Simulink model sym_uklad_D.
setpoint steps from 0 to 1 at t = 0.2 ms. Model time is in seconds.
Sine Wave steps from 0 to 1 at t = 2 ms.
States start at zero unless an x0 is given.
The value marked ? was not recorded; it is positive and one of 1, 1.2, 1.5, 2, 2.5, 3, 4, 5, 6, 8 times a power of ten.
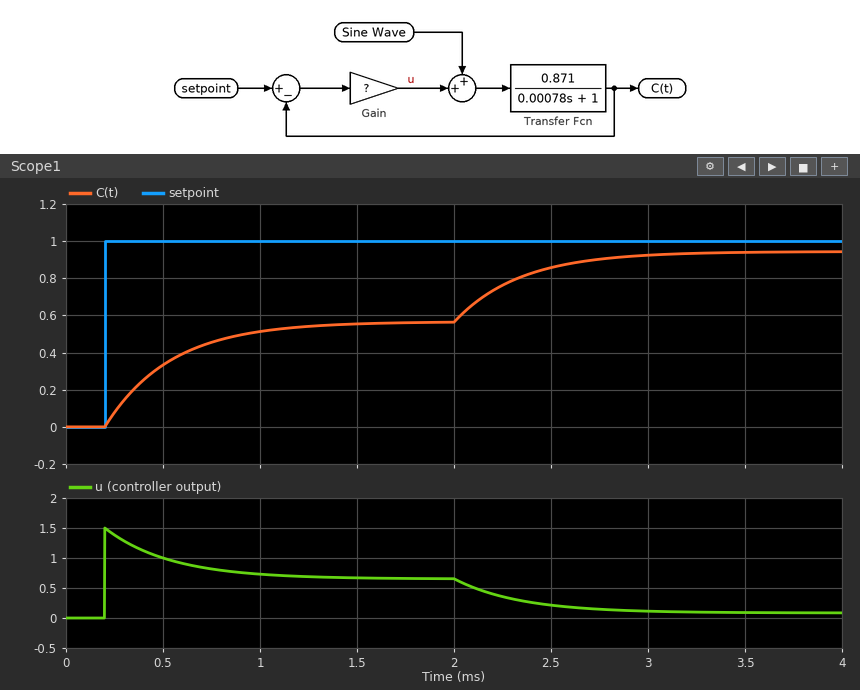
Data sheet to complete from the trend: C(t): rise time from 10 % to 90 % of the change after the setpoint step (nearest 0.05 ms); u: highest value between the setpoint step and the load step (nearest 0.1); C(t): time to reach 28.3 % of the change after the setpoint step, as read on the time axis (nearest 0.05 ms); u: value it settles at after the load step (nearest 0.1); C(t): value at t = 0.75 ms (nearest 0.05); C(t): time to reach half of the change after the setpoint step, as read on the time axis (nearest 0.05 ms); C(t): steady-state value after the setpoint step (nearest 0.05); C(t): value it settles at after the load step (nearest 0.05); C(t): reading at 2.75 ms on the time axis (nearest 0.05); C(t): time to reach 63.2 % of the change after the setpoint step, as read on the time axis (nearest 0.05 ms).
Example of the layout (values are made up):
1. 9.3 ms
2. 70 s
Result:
1. 0.75 ms
2. 1.5
3. 0.30 ms
4. 0.1
5. 0.45
6. 0.45 ms
7. 0.55
8. 0.95
9. 0.90
10. 0.55 ms
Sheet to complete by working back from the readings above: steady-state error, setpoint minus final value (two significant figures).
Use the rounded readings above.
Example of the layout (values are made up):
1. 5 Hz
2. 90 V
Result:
1. 0.45
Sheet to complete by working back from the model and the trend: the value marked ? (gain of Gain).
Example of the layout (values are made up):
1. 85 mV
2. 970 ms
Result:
1. 1.5
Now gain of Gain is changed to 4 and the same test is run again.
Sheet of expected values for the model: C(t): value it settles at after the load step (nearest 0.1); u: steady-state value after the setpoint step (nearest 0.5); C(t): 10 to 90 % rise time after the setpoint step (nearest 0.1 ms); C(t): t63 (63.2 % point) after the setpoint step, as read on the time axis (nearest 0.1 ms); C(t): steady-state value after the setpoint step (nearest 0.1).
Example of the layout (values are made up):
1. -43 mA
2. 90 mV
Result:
1. 1.0
2. 1.0
3. 0.4 ms
4. 0.4 ms
5. 0.8
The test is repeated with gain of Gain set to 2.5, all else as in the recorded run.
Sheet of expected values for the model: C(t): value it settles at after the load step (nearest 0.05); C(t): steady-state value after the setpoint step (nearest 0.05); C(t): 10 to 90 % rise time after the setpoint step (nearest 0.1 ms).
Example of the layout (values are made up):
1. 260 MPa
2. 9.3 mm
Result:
1. 0.95
2. 0.70
3. 0.5 ms
